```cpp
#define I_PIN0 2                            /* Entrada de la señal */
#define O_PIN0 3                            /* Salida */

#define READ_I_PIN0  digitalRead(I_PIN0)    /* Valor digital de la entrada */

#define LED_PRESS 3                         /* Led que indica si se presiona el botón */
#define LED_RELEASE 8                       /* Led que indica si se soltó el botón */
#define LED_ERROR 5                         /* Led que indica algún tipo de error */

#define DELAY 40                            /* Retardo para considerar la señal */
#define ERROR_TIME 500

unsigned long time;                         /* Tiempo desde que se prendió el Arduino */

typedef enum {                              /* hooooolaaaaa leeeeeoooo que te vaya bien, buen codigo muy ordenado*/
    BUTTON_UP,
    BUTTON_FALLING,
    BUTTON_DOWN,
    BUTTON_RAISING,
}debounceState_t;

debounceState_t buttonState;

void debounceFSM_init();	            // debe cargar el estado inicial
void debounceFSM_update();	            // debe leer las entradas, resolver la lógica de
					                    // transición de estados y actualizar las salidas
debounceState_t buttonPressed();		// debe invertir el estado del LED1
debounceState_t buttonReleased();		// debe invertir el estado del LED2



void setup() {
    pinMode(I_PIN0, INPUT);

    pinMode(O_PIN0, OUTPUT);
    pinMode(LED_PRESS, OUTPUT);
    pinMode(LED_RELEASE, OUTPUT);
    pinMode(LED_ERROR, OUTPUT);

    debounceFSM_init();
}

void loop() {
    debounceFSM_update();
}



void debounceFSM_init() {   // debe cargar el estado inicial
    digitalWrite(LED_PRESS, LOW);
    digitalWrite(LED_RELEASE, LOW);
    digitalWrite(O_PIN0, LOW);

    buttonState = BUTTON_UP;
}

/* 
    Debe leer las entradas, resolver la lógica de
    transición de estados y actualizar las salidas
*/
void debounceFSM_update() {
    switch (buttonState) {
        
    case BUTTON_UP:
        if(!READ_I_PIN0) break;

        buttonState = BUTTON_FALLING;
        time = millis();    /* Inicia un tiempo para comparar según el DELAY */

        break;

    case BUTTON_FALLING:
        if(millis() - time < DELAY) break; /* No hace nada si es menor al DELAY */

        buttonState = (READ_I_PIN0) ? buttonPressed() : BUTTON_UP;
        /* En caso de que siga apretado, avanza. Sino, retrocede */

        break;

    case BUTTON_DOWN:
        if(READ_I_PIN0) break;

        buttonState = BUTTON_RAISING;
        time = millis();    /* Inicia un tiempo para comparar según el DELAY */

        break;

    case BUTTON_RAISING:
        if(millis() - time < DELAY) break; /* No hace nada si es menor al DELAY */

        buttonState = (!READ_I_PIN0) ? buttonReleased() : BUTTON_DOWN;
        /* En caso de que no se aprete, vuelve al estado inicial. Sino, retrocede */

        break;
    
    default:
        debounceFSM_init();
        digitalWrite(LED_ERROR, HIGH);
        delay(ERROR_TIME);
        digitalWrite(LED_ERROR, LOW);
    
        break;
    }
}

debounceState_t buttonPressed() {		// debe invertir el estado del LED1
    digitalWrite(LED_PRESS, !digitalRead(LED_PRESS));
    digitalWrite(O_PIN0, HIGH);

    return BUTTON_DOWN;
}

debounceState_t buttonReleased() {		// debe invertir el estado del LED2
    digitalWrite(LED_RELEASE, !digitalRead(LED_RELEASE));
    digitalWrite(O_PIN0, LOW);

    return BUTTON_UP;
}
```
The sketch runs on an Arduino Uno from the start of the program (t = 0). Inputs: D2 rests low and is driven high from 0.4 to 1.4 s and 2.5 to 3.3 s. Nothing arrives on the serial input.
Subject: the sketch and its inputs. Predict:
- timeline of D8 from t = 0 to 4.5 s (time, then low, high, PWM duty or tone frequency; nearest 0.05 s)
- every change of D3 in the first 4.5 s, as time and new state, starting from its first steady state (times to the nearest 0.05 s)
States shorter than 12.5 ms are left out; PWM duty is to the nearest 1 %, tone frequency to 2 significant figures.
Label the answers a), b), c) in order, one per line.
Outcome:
a) 0 s low; 1.45 s high; 3.35 s low
b) 0 s low; 0.45 s high; 1.45 s low; 2.55 s high; 3.35 s low
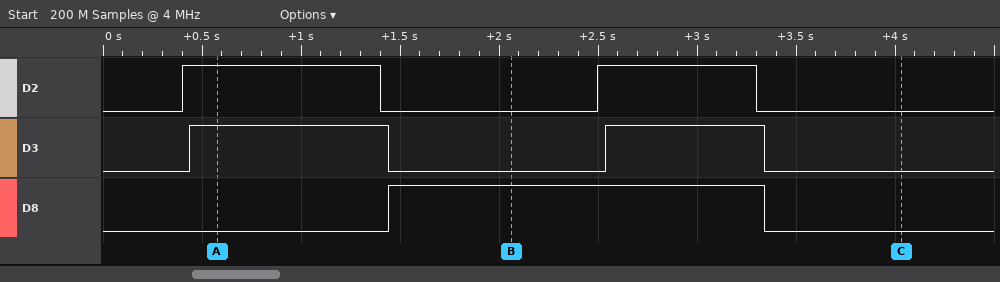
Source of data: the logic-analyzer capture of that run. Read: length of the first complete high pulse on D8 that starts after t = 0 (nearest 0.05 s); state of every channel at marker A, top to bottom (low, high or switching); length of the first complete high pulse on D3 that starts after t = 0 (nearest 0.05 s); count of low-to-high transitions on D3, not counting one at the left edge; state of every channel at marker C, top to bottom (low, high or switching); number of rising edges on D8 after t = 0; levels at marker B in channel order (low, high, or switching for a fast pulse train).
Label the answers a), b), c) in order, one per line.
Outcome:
a) 1.90 s
b) D2 high, D3 high, D8 low
c) 1.00 s
d) 2
e) D2 low, D3 low, D8 low
f) 1
g) D2 low, D3 low, D8 high
